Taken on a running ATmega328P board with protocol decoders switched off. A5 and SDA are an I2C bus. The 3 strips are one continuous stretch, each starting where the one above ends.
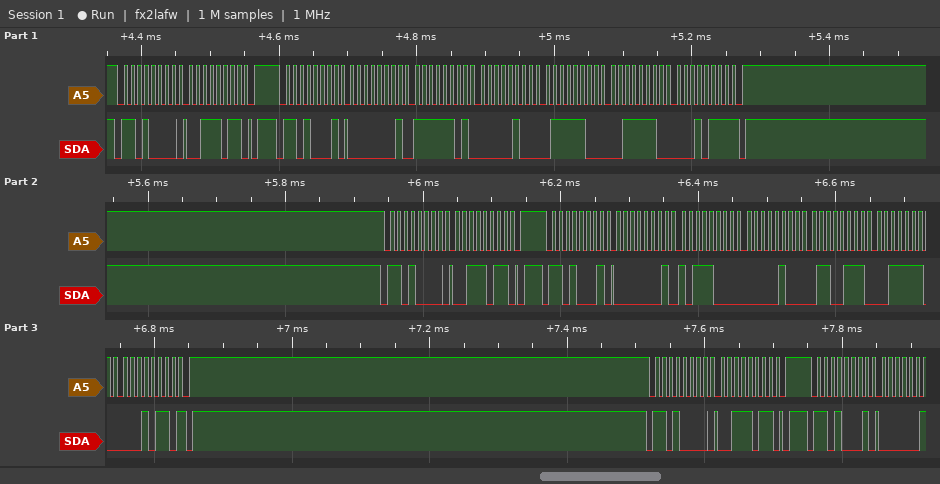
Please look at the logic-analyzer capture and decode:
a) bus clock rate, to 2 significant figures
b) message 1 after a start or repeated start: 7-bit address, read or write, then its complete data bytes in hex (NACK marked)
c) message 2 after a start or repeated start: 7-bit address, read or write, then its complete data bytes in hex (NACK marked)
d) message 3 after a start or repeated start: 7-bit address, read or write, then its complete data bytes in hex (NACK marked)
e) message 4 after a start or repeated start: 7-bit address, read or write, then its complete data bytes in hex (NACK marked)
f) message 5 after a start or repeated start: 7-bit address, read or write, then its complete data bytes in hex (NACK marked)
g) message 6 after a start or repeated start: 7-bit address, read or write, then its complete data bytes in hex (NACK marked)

100 kHz
0x68 write: 3B
0x68 read: 01 FD 04 7C 3E 17 NACK
0x68 write: 3B
0x68 read: 01 B8 04 67 3E 16 NACK
0x68 write: 3B
0x68 read
